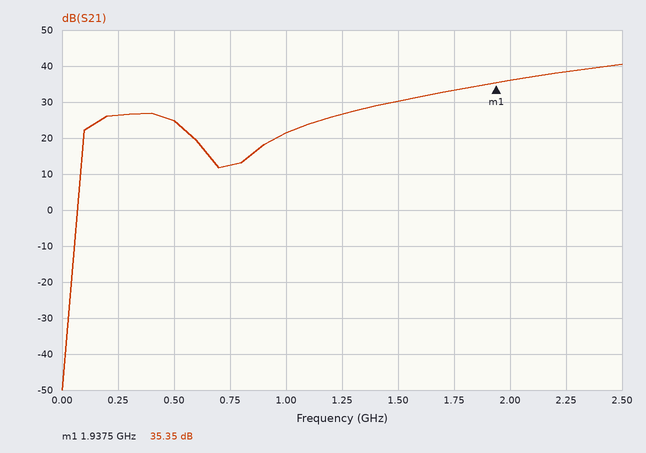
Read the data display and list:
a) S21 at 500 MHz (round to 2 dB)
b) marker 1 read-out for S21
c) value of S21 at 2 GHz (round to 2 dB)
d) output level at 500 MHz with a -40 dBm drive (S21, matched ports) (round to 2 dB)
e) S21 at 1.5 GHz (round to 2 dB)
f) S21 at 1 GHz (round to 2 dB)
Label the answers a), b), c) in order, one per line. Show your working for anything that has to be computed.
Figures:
a) 24 dB
b) 35.35 dB
c) 36 dB
d) -40 dBm + (24 dB) = -16 dBm
e) 30 dB
f) 22 dB
